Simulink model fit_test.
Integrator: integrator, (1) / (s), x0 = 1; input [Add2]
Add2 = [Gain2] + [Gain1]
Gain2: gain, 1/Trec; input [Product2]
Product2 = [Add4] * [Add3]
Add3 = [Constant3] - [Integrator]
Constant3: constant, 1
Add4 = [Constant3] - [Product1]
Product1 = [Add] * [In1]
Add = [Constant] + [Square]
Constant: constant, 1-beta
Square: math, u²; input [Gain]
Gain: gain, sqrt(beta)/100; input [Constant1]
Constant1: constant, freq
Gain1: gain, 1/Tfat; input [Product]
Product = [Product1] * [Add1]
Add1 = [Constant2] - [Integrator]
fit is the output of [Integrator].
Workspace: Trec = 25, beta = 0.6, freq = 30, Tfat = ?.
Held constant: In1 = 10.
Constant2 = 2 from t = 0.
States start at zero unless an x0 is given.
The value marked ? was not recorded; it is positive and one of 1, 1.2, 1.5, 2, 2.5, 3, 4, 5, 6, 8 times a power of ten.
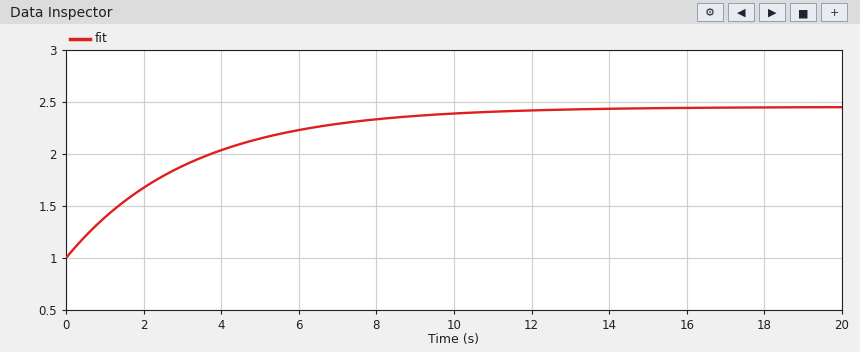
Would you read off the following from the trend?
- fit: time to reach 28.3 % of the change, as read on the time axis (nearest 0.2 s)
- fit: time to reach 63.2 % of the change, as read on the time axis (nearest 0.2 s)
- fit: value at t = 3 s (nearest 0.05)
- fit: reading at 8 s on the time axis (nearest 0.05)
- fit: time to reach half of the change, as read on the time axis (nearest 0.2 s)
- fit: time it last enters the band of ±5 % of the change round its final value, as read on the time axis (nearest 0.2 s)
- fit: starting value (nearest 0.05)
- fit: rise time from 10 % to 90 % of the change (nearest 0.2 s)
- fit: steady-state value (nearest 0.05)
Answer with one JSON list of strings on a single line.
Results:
["1.0 s", "3.2 s", "1.90", "2.35", "2.2 s", "9.6 s", "1.00", "7.0 s", "2.45"]
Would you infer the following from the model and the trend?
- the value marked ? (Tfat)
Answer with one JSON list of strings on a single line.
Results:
["10"]
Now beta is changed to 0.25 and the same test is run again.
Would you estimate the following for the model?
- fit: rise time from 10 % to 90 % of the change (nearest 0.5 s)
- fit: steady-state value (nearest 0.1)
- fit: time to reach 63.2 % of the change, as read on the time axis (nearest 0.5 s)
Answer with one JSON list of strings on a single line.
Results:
["4.5 s", "2.5", "2.0 s"]
